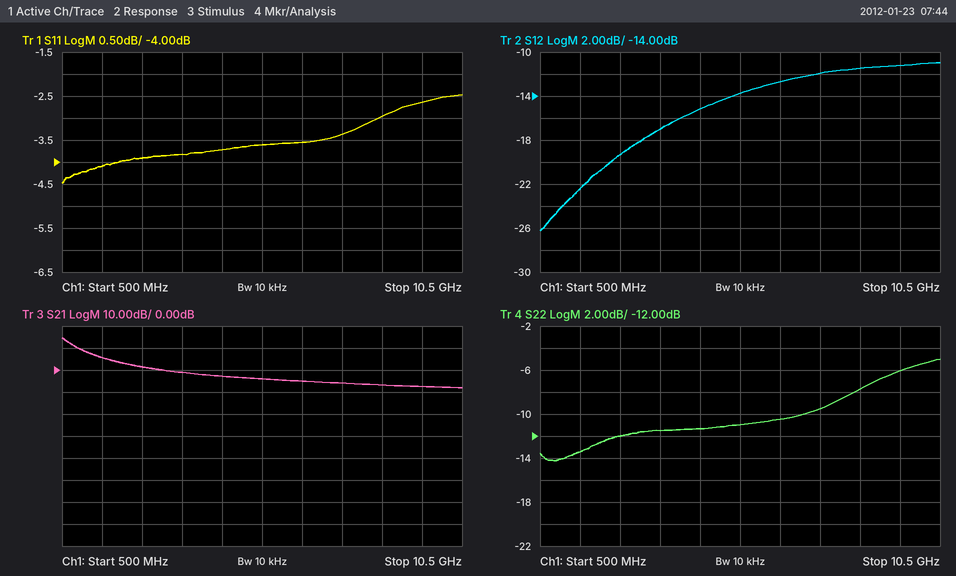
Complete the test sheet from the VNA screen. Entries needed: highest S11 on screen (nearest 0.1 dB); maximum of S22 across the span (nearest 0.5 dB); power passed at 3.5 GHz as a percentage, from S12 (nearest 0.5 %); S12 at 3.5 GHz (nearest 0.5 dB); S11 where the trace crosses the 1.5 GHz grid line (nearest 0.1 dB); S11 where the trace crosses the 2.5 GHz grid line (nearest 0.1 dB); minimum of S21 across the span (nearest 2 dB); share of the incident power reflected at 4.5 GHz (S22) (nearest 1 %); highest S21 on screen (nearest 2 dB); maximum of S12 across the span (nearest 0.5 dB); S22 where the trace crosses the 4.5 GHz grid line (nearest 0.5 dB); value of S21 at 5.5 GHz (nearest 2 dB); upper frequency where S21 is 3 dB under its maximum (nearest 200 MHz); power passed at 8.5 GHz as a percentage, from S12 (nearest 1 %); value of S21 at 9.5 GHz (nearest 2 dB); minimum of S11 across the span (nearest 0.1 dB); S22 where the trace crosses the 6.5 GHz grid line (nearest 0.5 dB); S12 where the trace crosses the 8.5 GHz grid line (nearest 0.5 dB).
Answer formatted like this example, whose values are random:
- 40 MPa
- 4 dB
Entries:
- -2.5 dB
- -5.0 dB
- 2.0 %
- -17.0 dB
- -4.1 dB
- -3.9 dB
- -8 dB
- 7 %
- 14 dB
- -11.0 dB
- -11.5 dB
- -4 dB
- 800 MHz
- 7 %
- -8 dB
- -4.5 dB
- -10.5 dB
- -11.5 dB
